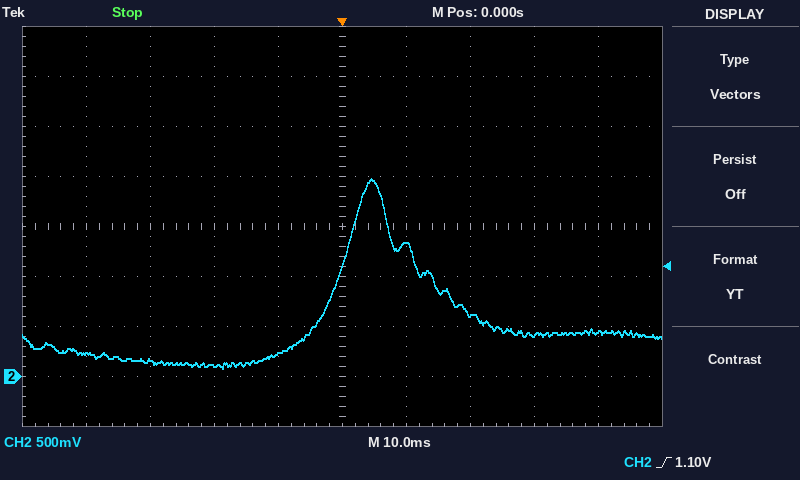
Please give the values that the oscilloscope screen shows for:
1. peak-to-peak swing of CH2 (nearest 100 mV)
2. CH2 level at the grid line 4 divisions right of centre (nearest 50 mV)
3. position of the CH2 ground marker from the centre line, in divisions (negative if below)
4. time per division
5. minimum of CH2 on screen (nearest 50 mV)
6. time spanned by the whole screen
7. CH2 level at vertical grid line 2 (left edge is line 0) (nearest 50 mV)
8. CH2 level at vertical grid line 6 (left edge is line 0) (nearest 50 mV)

1.90 V
450 mV
-3.0 div
10 ms
100 mV
100 ms
150 mV
1.35 V
